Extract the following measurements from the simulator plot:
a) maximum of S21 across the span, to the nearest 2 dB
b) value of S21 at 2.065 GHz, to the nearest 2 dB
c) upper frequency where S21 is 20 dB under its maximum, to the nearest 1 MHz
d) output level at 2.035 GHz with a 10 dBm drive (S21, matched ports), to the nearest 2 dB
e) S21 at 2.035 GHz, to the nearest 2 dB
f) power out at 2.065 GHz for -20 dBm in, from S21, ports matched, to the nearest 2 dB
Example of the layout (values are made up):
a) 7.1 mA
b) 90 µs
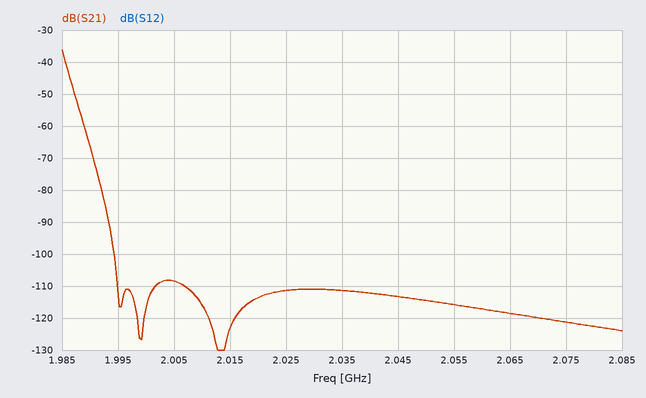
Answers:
a) -36 dB
b) -118 dB
c) 1.988 GHz
d) -102 dBm
e) -112 dB
f) -138 dBm
